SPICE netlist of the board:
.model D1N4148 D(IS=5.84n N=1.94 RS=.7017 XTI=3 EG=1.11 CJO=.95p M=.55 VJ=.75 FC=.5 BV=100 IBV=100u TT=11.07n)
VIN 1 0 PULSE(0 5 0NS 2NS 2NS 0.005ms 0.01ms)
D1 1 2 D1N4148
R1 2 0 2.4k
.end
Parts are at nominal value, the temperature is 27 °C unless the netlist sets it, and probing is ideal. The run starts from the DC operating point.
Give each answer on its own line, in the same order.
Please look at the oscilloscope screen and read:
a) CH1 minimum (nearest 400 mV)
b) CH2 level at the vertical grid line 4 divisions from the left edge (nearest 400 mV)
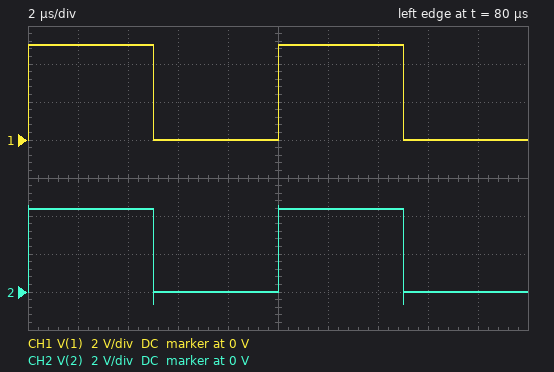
0 V
0 V
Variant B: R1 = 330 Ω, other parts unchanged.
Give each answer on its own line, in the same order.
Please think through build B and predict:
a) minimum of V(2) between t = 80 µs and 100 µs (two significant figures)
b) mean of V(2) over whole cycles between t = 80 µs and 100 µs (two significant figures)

-730 mV
2.1 V
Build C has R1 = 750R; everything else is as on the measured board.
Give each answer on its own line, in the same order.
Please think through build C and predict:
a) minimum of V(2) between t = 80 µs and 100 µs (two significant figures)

-690 mV
